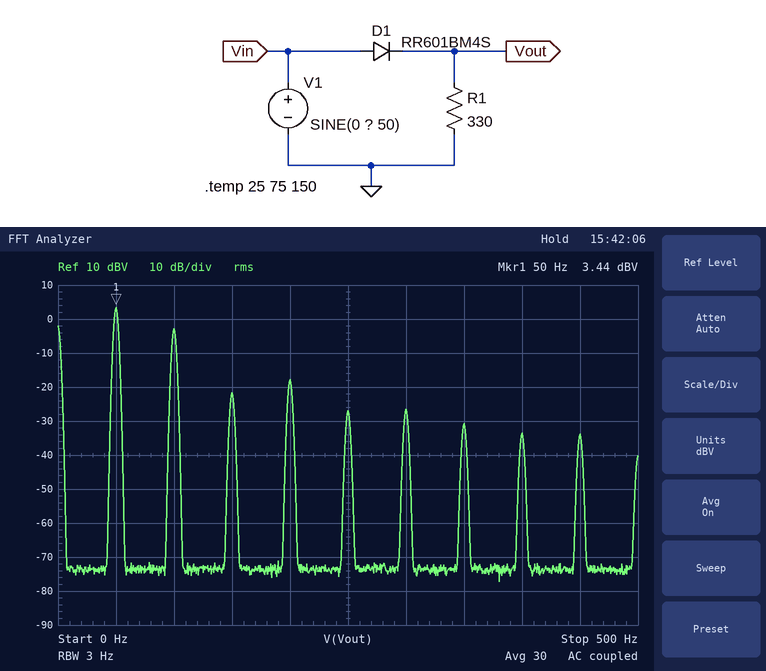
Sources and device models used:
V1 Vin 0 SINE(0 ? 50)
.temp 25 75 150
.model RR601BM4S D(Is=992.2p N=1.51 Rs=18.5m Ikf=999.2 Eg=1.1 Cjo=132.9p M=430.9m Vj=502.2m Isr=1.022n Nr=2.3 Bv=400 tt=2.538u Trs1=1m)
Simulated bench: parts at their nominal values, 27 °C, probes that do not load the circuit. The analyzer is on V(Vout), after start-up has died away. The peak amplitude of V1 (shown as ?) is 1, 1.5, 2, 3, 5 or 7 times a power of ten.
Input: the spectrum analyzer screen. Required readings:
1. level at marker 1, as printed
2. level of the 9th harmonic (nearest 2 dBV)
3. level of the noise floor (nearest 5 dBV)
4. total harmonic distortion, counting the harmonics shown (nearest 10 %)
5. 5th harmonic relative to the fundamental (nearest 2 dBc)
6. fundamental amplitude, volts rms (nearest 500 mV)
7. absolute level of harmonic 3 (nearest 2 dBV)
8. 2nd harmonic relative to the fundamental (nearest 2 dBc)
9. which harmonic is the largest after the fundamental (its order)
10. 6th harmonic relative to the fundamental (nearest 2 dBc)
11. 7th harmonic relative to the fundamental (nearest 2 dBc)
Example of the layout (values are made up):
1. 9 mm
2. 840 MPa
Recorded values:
1. 3.44 dBV
2. -34 dBV
3. -75 dBV
4. 50 %
5. -30 dBc
6. 1.5 V
7. -22 dBV
8. -6 dBc
9. 2
10. -30 dBc
11. -34 dBc
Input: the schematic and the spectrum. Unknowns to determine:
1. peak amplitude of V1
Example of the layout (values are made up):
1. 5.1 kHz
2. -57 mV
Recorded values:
1. 5 V
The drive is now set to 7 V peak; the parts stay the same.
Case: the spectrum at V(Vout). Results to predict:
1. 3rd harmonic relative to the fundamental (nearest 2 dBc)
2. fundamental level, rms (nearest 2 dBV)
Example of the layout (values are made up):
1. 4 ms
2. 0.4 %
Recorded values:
1. -28 dBc
2. 6 dBV
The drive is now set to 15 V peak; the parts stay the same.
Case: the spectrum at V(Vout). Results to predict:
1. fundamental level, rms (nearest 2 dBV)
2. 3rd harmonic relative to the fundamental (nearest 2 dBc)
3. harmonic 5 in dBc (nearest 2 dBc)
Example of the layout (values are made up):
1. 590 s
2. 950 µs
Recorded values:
1. 14 dBV
2. -34 dBc
3. -40 dBc
